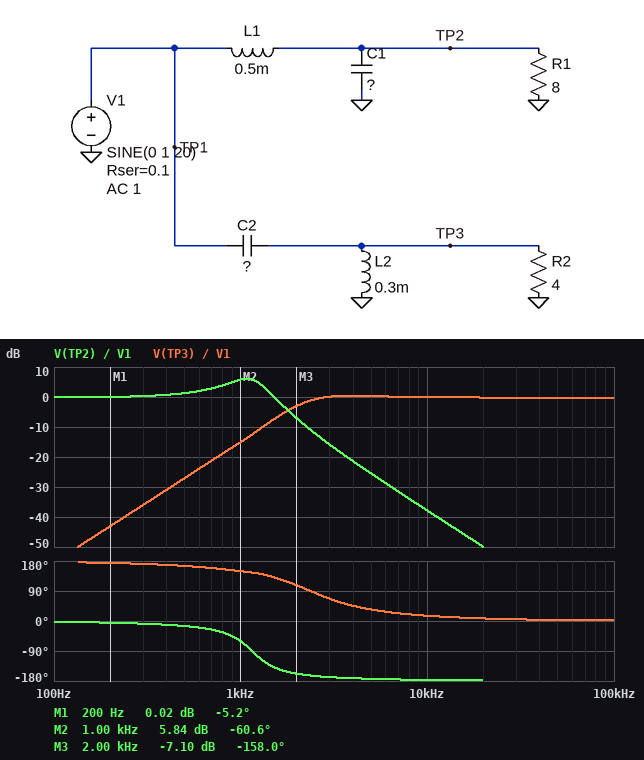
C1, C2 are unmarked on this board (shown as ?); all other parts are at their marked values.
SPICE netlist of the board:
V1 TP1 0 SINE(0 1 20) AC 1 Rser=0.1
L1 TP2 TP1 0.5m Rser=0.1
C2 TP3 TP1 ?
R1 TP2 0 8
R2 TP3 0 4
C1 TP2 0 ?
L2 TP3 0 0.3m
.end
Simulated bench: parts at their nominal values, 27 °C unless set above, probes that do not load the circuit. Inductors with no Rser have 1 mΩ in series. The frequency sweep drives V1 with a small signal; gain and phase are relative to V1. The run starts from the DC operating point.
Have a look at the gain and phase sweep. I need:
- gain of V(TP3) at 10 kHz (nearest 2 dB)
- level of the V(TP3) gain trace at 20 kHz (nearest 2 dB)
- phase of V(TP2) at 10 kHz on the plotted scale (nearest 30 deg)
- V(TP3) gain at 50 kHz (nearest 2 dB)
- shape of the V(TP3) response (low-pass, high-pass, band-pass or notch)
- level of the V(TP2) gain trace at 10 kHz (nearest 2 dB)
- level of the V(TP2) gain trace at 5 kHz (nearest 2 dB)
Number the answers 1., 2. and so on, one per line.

1. 0 dB
2. 0 dB
3. -180 deg
4. 0 dB
5. high-pass
6. -38 dB
7. -26 dB
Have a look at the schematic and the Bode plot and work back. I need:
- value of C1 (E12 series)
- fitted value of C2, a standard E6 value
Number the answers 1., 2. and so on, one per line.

1. 39 µF
2. 15 µF
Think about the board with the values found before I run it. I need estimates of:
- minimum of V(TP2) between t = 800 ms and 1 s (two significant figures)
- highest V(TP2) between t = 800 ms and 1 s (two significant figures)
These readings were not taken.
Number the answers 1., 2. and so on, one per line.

1. -980 mV
2. 980 mV
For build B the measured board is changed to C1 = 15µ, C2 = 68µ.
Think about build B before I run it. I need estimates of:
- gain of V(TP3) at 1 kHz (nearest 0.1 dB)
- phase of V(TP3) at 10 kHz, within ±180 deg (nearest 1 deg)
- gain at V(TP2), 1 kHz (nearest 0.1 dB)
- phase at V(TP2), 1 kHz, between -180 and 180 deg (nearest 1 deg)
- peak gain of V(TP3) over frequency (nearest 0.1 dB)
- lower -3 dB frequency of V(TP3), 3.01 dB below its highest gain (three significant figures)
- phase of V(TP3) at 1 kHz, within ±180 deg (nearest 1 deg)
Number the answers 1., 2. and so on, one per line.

1. 3.3 dB
2. 4 deg
3. 1.0 dB
4. -33 deg
5. 4.9 dB
6. 935 Hz
7. 109 deg
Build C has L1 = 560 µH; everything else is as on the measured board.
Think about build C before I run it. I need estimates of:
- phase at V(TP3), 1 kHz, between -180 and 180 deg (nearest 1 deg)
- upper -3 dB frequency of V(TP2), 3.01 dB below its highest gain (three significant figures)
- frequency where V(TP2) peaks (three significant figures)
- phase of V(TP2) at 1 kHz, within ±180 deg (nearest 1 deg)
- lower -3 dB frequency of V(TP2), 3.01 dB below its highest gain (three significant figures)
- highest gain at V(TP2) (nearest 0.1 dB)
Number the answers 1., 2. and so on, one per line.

1. 150 deg
2. 1.27 kHz
3. 1.01 kHz
4. -72 deg
5. 656 Hz
6. 5.8 dB
